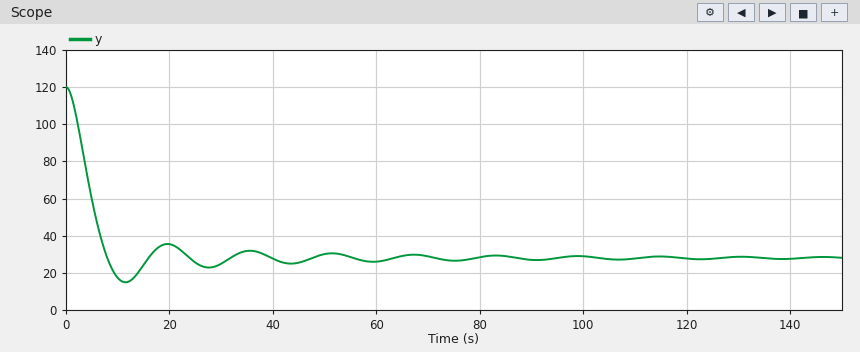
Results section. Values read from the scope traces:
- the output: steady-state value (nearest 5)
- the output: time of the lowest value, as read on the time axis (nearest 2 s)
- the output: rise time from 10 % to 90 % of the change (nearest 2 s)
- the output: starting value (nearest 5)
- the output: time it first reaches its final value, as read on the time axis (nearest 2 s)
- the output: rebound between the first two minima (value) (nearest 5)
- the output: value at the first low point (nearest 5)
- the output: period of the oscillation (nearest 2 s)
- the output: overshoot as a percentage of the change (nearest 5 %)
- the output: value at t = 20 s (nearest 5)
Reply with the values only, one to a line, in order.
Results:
30
12 s
6 s
120
8 s
35
15
16 s
15 %
35
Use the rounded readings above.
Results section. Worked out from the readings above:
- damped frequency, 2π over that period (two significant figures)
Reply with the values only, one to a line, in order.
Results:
0.39 rad/s
